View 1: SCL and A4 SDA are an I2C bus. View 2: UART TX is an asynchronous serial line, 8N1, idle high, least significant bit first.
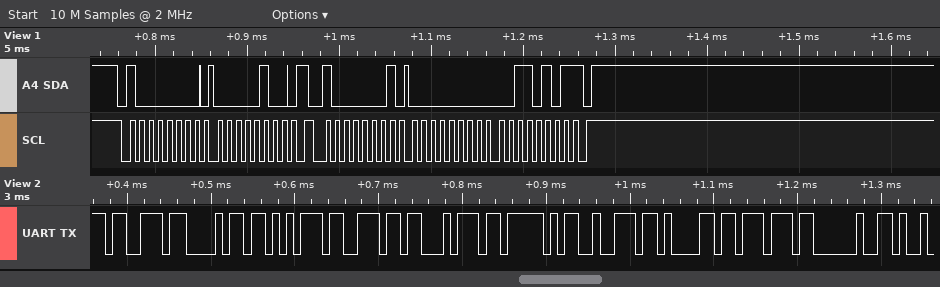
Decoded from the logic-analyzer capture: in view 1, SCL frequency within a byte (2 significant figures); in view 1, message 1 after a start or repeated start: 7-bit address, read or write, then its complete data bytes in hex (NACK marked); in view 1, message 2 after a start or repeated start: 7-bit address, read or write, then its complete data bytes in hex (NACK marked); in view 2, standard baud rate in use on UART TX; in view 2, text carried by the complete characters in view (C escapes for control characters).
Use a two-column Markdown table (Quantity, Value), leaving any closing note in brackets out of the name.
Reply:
| Quantity | Value |
|---|---|
| in view 1, SCL frequency within a byte | 100 kHz |
| in view 1, message 1 after a start or repeated start: 7-bit address, read or write, then its complete data bytes in hex | 0x40 write: 04 |
| in view 1, message 2 after a start or repeated start: 7-bit address, read or write, then its complete data bytes in hex | 0x40 read: 00 35 NACK |
| in view 2, standard baud rate in use on UART TX | 115200 baud |
| in view 2, text carried by the complete characters in view | "shunt_raw " |
